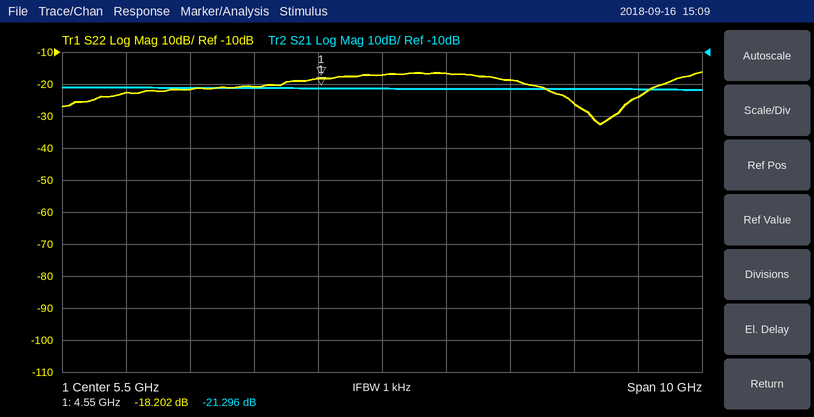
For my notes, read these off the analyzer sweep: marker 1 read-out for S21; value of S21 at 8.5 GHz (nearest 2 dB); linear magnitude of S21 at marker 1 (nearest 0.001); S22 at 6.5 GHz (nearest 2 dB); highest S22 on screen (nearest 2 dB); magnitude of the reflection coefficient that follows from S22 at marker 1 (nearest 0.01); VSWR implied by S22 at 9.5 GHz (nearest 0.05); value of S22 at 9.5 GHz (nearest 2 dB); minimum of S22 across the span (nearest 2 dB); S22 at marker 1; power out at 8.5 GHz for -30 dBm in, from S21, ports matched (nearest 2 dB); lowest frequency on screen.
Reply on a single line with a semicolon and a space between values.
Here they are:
-21.296 dB; -22 dB; 0.086; -16 dB; -16 dB; 0.12; 1.15; -24 dB; -32 dB; -18.202 dB; -52 dBm; 500 MHz
